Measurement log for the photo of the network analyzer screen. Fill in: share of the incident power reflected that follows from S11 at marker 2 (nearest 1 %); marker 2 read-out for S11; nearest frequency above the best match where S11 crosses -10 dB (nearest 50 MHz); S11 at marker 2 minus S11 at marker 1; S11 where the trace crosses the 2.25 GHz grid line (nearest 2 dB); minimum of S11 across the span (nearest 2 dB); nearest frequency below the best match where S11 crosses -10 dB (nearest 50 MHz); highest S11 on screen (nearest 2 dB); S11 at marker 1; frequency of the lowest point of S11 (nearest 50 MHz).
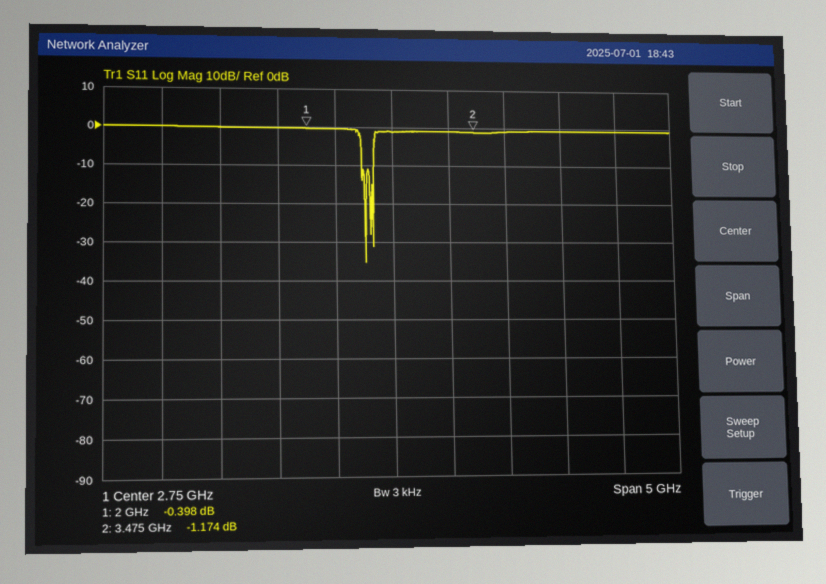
76 %
-1.174 dB
2.60 GHz
-0.776 dB
0 dB
-36 dB
2.50 GHz
0 dB
-0.398 dB
2.50 GHz
